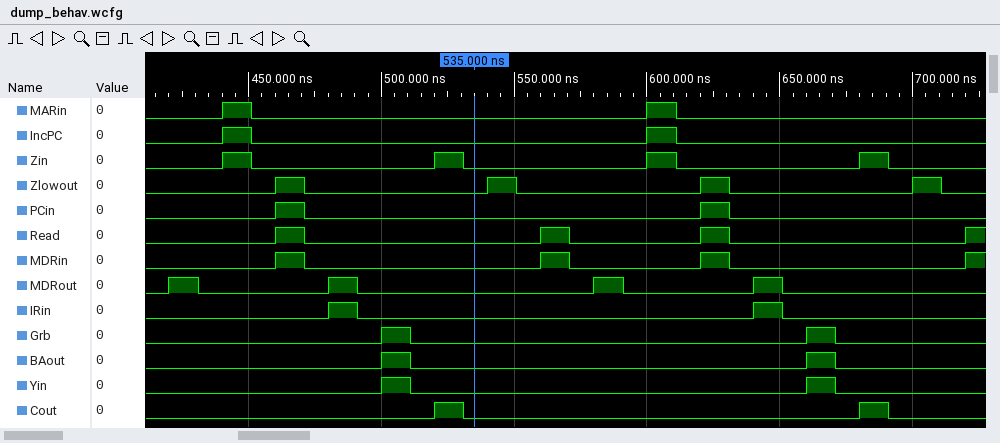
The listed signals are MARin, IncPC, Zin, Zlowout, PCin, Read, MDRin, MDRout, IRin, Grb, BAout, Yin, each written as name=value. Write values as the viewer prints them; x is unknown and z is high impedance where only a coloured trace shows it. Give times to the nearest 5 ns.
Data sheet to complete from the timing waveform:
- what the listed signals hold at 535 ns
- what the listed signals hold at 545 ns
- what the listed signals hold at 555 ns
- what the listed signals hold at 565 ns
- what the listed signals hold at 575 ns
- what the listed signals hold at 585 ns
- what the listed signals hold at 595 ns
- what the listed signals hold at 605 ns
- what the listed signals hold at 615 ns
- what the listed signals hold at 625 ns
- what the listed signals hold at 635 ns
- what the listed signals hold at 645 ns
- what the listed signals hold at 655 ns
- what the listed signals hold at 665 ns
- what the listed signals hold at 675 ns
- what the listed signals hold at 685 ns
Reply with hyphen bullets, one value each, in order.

- MARin=0, IncPC=0, Zin=0, Zlowout=0, PCin=0, Read=0, MDRin=0, MDRout=0, IRin=0, Grb=0, BAout=0, Yin=0
- MARin=0, IncPC=0, Zin=0, Zlowout=1, PCin=0, Read=0, MDRin=0, MDRout=0, IRin=0, Grb=0, BAout=0, Yin=0
- MARin=0, IncPC=0, Zin=0, Zlowout=0, PCin=0, Read=0, MDRin=0, MDRout=0, IRin=0, Grb=0, BAout=0, Yin=0
- MARin=0, IncPC=0, Zin=0, Zlowout=0, PCin=0, Read=1, MDRin=1, MDRout=0, IRin=0, Grb=0, BAout=0, Yin=0
- MARin=0, IncPC=0, Zin=0, Zlowout=0, PCin=0, Read=0, MDRin=0, MDRout=0, IRin=0, Grb=0, BAout=0, Yin=0
- MARin=0, IncPC=0, Zin=0, Zlowout=0, PCin=0, Read=0, MDRin=0, MDRout=1, IRin=0, Grb=0, BAout=0, Yin=0
- MARin=0, IncPC=0, Zin=0, Zlowout=0, PCin=0, Read=0, MDRin=0, MDRout=0, IRin=0, Grb=0, BAout=0, Yin=0
- MARin=1, IncPC=1, Zin=1, Zlowout=0, PCin=0, Read=0, MDRin=0, MDRout=0, IRin=0, Grb=0, BAout=0, Yin=0
- MARin=0, IncPC=0, Zin=0, Zlowout=0, PCin=0, Read=0, MDRin=0, MDRout=0, IRin=0, Grb=0, BAout=0, Yin=0
- MARin=0, IncPC=0, Zin=0, Zlowout=1, PCin=1, Read=1, MDRin=1, MDRout=0, IRin=0, Grb=0, BAout=0, Yin=0
- MARin=0, IncPC=0, Zin=0, Zlowout=0, PCin=0, Read=0, MDRin=0, MDRout=0, IRin=0, Grb=0, BAout=0, Yin=0
- MARin=0, IncPC=0, Zin=0, Zlowout=0, PCin=0, Read=0, MDRin=0, MDRout=1, IRin=1, Grb=0, BAout=0, Yin=0
- MARin=0, IncPC=0, Zin=0, Zlowout=0, PCin=0, Read=0, MDRin=0, MDRout=0, IRin=0, Grb=0, BAout=0, Yin=0
- MARin=0, IncPC=0, Zin=0, Zlowout=0, PCin=0, Read=0, MDRin=0, MDRout=0, IRin=0, Grb=1, BAout=1, Yin=1
- MARin=0, IncPC=0, Zin=0, Zlowout=0, PCin=0, Read=0, MDRin=0, MDRout=0, IRin=0, Grb=0, BAout=0, Yin=0
- MARin=0, IncPC=0, Zin=1, Zlowout=0, PCin=0, Read=0, MDRin=0, MDRout=0, IRin=0, Grb=0, BAout=0, Yin=0
